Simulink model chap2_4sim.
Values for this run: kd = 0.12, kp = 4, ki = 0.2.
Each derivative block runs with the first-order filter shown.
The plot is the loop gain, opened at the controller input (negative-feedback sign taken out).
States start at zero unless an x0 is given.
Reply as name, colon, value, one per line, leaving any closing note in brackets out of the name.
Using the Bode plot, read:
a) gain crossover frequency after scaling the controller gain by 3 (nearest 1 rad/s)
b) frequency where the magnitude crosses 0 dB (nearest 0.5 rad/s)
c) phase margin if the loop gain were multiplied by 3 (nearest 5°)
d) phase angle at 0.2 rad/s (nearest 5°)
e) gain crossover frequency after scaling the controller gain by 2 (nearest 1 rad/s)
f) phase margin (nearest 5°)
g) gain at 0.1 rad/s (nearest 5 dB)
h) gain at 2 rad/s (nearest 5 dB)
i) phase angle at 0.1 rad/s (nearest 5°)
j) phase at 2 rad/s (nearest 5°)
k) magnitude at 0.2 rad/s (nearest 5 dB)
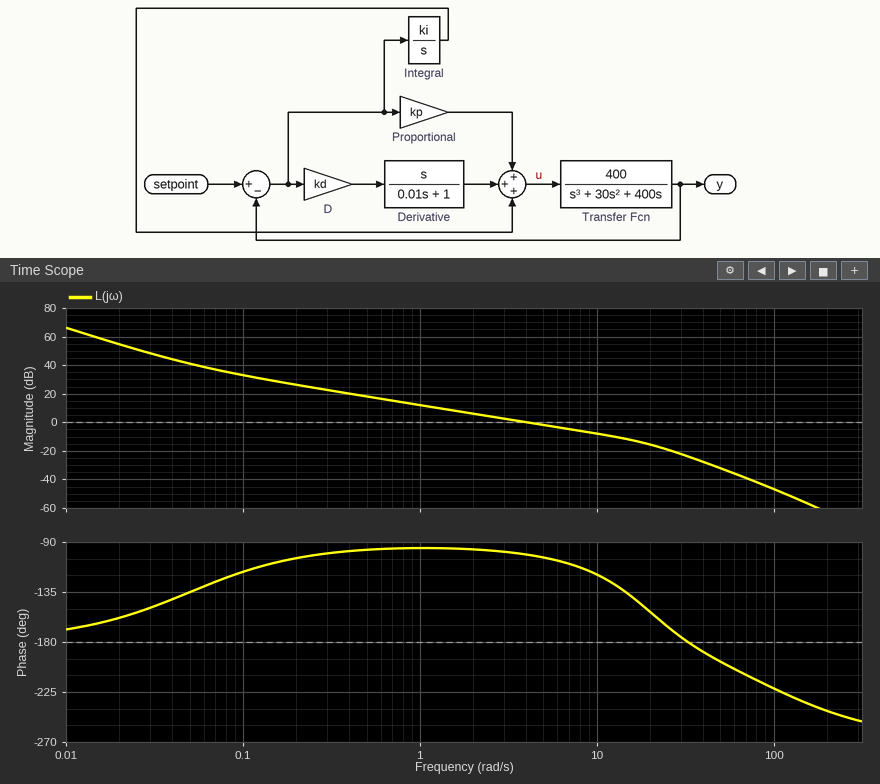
gain crossover frequency after scaling the controller gain by 3: 12 rad/s
frequency where the magnitude crosses 0 dB: 4.0 rad/s
phase margin if the loop gain were multiplied by 3: 55°
phase angle at 0.2 rad/s: -105°
gain crossover frequency after scaling the controller gain by 2: 8 rad/s
phase margin: 80°
gain at 0.1 rad/s: 35 dB
gain at 2 rad/s: 5 dB
phase angle at 0.1 rad/s: -115°
phase at 2 rad/s: -95°
magnitude at 0.2 rad/s: 25 dB
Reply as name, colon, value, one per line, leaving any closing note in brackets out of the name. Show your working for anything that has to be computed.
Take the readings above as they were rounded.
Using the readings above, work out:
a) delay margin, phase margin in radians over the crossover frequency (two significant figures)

delay margin, phase margin in radians over the crossover frequency: 80 × π / 180 / 4 = 0.35 s
